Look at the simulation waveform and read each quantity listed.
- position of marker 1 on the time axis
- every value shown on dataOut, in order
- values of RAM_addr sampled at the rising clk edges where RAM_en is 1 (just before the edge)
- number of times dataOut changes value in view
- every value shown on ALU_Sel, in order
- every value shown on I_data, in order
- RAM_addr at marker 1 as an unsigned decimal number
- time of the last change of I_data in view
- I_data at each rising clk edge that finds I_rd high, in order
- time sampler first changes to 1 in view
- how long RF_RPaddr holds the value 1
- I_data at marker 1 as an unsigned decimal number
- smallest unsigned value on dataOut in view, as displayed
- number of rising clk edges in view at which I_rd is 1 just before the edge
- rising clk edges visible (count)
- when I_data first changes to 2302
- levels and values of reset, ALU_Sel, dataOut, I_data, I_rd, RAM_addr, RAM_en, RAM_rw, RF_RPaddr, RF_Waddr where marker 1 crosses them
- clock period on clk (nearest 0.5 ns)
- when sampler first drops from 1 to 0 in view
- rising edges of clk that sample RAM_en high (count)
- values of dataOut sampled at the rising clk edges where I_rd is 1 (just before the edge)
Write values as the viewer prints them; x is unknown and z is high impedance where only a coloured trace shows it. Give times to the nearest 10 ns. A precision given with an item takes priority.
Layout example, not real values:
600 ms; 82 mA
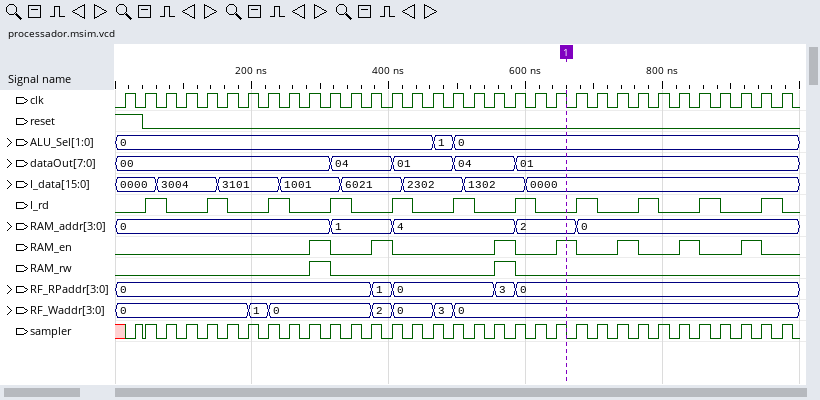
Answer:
660 ns; 00, 04, 01, 04, 01; 0, 1, 4, 2, 0, 0, 0; 4; 0, 1, 0; 0000, 3004, 3101, 1001, 6021, 2302, 1302, 0000; 2; 600 ns; 3004, 3101, 1001, 6021, 2302, 1302, 0000, 0000, 0000, 0000, 0000; 30 ns; 30 ns; 0; 00; 11; 33; 420 ns; reset=0, ALU_Sel=0, dataOut=01, I_data=0000, I_rd=0, RAM_addr=2, RAM_en=1, RAM_rw=0, RF_RPaddr=0, RF_Waddr=0; 30 ns; 40 ns; 7; 00, 00, 00, 04, 01, 04, 01, 01, 01, 01, 01
